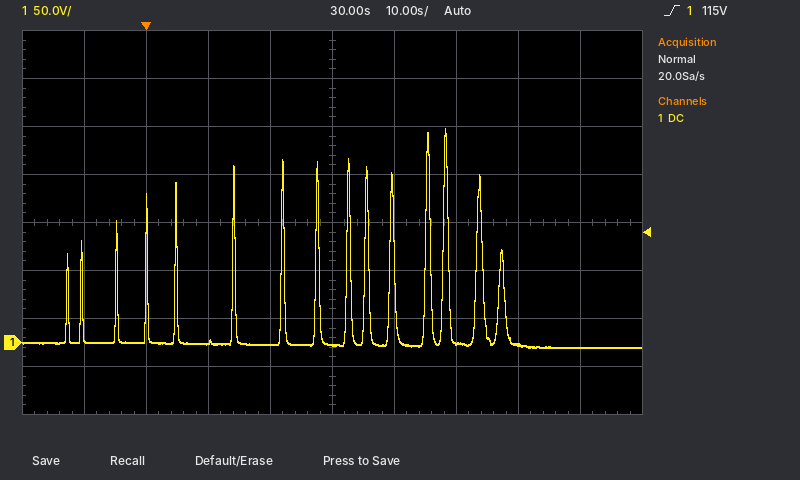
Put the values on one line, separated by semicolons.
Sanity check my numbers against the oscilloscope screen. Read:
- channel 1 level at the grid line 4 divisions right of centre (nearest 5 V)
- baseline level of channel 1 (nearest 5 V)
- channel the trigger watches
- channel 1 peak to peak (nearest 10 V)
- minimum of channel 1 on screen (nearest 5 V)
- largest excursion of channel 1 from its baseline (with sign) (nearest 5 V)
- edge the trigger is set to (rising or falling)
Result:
-5 V; 0 V; channel 1; 230 V; -5 V; +225 V; rising
